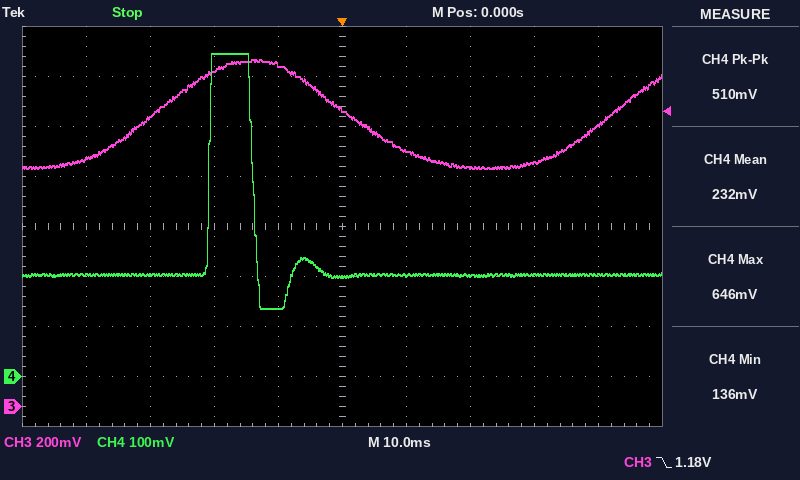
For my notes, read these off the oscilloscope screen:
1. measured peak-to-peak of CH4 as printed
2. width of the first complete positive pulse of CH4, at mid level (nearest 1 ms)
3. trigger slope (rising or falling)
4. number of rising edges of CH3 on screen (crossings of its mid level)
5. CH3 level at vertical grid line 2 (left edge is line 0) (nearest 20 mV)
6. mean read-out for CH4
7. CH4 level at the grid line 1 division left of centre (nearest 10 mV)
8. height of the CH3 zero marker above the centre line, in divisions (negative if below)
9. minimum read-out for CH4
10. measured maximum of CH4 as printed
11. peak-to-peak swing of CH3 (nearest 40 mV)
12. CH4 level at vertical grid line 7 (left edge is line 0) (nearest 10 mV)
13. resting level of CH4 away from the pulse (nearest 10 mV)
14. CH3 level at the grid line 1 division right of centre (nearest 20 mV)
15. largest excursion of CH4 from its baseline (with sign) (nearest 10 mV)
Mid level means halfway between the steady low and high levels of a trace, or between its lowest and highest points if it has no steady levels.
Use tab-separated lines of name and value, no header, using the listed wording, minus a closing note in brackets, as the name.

measured peak-to-peak of CH4 as printed	510 mV
width of the first complete positive pulse of CH4, at mid level	7 ms
trigger slope	falling
number of rising edges of CH3 on screen	2
CH3 level at vertical grid line 2 (left edge is line 0)	1.16 V
mean read-out for CH4	232 mV
CH4 level at the grid line 1 division left of centre	140 mV
height of the CH3 zero marker above the centre line, in divisions	-3.6 div
minimum read-out for CH4	136 mV
measured maximum of CH4 as printed	646 mV
peak-to-peak swing of CH3	440 mV
CH4 level at vertical grid line 7 (left edge is line 0)	200 mV
resting level of CH4 away from the pulse	200 mV
CH3 level at the grid line 1 division right of centre	1.02 V
largest excursion of CH4 from its baseline (with sign)	+440 mV
